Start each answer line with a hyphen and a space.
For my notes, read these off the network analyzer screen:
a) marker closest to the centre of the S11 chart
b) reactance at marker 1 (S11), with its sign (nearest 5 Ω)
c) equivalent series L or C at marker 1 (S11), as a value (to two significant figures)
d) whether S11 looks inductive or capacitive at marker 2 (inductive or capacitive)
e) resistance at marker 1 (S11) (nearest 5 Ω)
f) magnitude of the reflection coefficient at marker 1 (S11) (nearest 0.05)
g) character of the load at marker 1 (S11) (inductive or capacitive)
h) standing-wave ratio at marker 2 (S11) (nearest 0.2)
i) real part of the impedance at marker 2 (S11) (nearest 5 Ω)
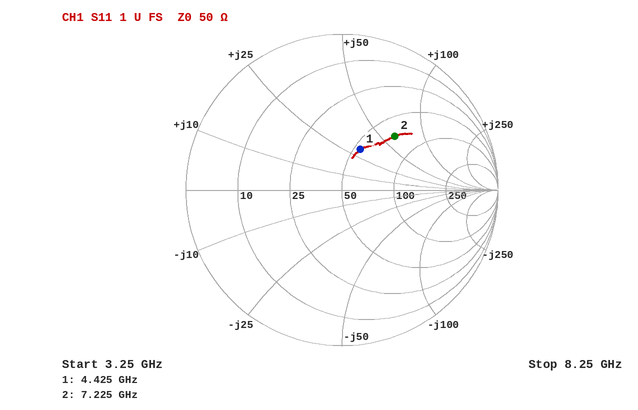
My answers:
- marker 1
- +30 Ω
- 1.1 nH
- inductive
- 55 Ω
- 0.30
- inductive
- 2.8
- 70 Ω
